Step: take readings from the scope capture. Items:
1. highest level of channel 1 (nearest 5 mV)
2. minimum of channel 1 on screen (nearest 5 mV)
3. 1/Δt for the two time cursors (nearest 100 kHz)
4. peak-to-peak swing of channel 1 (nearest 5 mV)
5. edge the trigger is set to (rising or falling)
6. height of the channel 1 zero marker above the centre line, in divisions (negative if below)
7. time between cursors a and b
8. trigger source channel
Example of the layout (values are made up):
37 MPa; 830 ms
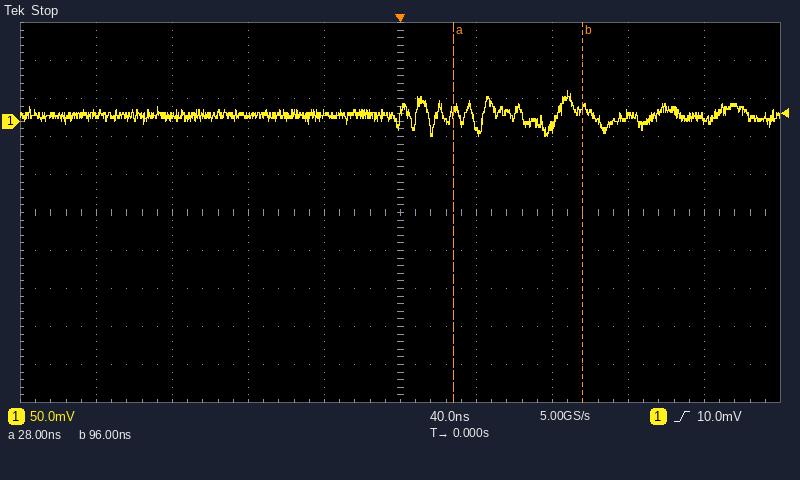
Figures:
40 mV; -20 mV; 14.7 MHz; 60 mV; rising; +2.4 div; 68 ns; channel 1
